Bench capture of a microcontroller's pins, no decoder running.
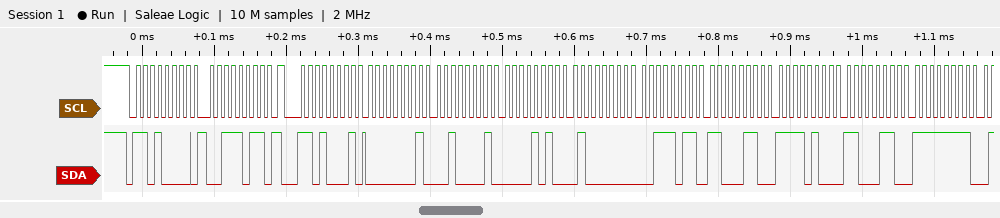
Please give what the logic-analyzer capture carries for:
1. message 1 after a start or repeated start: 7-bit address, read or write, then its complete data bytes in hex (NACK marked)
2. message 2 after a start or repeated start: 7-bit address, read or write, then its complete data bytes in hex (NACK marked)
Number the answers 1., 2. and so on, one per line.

1. 0x68 write: 3B
2. 0x68 read: 01 21 0A 40 3B C6 F4 C6 FF
